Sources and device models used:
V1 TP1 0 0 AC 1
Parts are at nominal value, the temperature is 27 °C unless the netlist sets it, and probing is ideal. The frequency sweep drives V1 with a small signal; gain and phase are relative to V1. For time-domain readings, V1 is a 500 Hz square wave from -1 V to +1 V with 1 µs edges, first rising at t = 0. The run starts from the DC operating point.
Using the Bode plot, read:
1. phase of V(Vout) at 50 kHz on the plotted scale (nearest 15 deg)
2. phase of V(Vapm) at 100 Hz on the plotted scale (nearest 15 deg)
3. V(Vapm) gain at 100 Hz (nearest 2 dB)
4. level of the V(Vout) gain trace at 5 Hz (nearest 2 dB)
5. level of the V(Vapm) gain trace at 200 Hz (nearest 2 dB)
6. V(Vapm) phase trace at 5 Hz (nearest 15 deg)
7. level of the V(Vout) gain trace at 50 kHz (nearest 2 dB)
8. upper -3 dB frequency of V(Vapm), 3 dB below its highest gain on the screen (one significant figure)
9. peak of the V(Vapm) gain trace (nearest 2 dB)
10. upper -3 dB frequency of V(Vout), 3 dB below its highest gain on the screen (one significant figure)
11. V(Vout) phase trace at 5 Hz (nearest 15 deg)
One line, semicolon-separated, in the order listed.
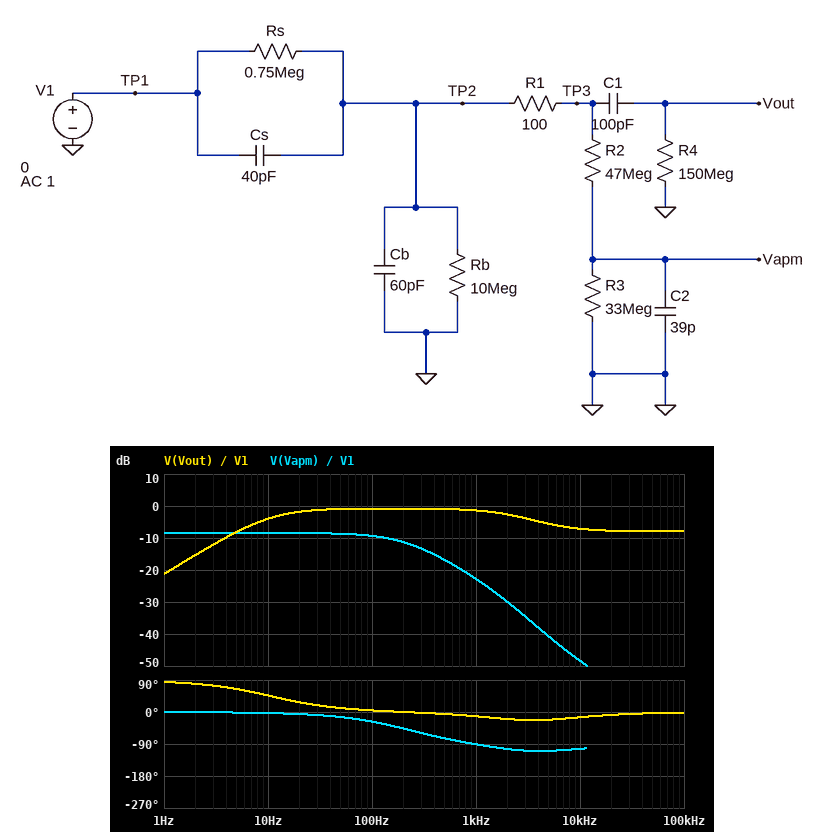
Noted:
0 deg; -30 deg; -10 dB; -8 dB; -12 dB; 0 deg; -8 dB; 200 Hz; -8 dB; 3 kHz; 60 deg
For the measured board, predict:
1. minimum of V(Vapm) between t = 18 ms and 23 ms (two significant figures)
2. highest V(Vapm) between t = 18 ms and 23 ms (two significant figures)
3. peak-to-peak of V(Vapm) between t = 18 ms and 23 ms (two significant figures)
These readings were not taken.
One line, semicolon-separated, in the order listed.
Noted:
-210 mV; 210 mV; 420 mV
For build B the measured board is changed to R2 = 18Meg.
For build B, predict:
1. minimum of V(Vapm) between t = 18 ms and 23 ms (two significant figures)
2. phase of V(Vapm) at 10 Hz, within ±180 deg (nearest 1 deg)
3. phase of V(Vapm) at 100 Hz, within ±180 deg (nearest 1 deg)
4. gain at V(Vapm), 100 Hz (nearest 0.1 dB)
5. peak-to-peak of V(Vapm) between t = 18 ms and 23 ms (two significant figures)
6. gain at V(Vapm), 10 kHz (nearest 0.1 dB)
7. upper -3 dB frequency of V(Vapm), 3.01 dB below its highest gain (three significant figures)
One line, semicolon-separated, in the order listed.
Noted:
-460 mV; -2 deg; -18 deg; -4.9 dB; 910 mV; -40.0 dB; 332 Hz
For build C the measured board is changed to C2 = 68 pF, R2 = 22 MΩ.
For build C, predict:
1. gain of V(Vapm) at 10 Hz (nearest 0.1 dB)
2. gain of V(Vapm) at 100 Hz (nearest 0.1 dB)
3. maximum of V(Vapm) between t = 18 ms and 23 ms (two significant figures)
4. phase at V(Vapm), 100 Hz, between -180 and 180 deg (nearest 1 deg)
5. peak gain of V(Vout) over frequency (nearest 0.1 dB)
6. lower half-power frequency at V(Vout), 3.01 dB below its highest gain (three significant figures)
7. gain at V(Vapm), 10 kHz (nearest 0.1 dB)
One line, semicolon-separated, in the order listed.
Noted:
-5.2 dB; -6.5 dB; 260 mV; -31 deg; -0.9 dB; 10.3 Hz; -46.6 dB
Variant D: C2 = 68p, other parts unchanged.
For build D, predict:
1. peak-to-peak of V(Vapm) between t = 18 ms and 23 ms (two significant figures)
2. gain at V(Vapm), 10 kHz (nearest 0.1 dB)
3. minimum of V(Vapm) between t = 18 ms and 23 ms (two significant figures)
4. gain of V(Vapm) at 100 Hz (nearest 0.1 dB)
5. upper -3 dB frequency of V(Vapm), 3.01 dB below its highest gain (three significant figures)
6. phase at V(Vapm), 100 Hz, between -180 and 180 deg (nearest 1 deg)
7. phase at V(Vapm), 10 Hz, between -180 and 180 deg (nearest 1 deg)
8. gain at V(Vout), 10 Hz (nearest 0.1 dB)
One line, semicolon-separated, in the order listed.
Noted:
260 mV; -53.2 dB; -130 mV; -10.7 dB; 119 Hz; -41 deg; -5 deg; -4.0 dB
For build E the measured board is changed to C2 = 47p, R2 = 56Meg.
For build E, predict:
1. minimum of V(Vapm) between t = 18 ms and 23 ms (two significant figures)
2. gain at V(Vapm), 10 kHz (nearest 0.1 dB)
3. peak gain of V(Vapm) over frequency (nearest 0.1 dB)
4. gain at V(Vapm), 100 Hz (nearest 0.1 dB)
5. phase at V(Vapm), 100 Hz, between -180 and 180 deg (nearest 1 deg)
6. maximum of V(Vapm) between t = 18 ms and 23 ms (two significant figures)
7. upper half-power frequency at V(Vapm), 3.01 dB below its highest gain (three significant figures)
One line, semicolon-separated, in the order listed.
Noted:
-150 mV; -51.5 dB; -9.3 dB; -10.8 dB; -33 deg; 150 mV; 160 Hz
